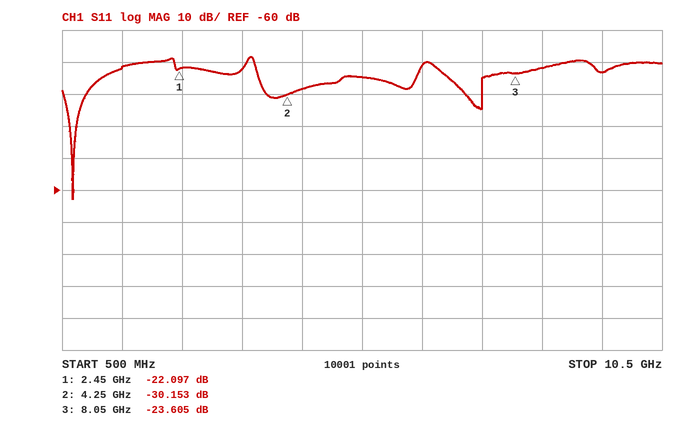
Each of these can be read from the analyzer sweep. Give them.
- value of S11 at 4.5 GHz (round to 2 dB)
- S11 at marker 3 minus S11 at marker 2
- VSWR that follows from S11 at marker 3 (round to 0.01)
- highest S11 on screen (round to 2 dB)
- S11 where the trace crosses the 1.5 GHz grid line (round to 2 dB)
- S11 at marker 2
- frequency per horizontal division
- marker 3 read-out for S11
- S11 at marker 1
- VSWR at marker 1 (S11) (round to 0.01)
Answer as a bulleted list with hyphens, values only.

- -28 dB
- 6.548 dB
- 1.14
- -18 dB
- -22 dB
- -30.153 dB
- 1 GHz
- -23.605 dB
- -22.097 dB
- 1.17
